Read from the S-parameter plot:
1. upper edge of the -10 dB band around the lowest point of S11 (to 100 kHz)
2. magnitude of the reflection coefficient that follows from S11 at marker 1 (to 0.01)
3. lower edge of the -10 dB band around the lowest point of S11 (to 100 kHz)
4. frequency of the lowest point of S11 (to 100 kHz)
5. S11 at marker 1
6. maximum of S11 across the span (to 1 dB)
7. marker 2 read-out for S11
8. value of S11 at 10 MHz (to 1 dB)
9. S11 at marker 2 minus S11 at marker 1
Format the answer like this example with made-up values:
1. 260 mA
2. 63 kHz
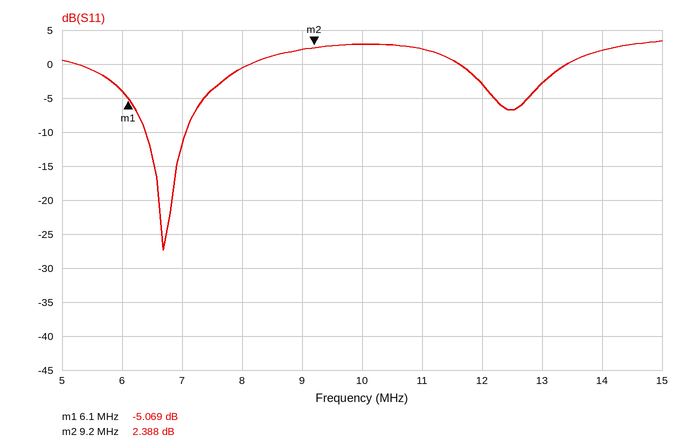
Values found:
1. 7.1 MHz
2. 0.56
3. 6.4 MHz
4. 6.7 MHz
5. -5.069 dB
6. 3 dB
7. 2.388 dB
8. 3 dB
9. 7.457 dB
